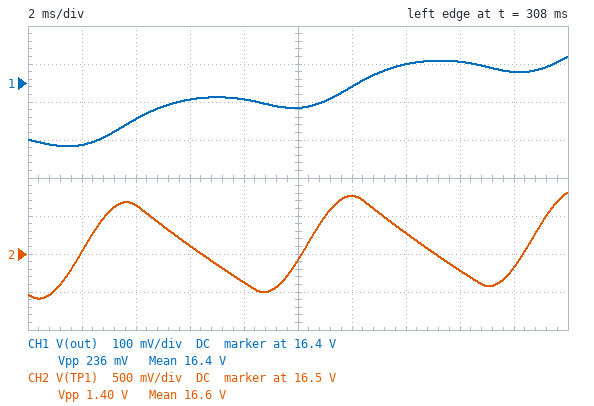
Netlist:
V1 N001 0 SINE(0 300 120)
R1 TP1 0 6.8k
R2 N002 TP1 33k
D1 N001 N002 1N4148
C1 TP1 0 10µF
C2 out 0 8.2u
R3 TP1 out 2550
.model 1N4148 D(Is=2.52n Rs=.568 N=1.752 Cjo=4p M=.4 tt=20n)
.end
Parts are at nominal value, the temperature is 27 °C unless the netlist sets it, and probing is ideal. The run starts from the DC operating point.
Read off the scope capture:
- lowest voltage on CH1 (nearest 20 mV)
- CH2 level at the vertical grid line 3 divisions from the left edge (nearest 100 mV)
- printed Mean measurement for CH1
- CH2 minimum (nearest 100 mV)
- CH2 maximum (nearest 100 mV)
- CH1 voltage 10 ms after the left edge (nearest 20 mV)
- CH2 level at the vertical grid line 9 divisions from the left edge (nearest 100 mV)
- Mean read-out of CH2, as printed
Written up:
16.24 V
16.6 V
16.4 V
15.9 V
17.3 V
16.34 V
16.3 V
16.6 V
